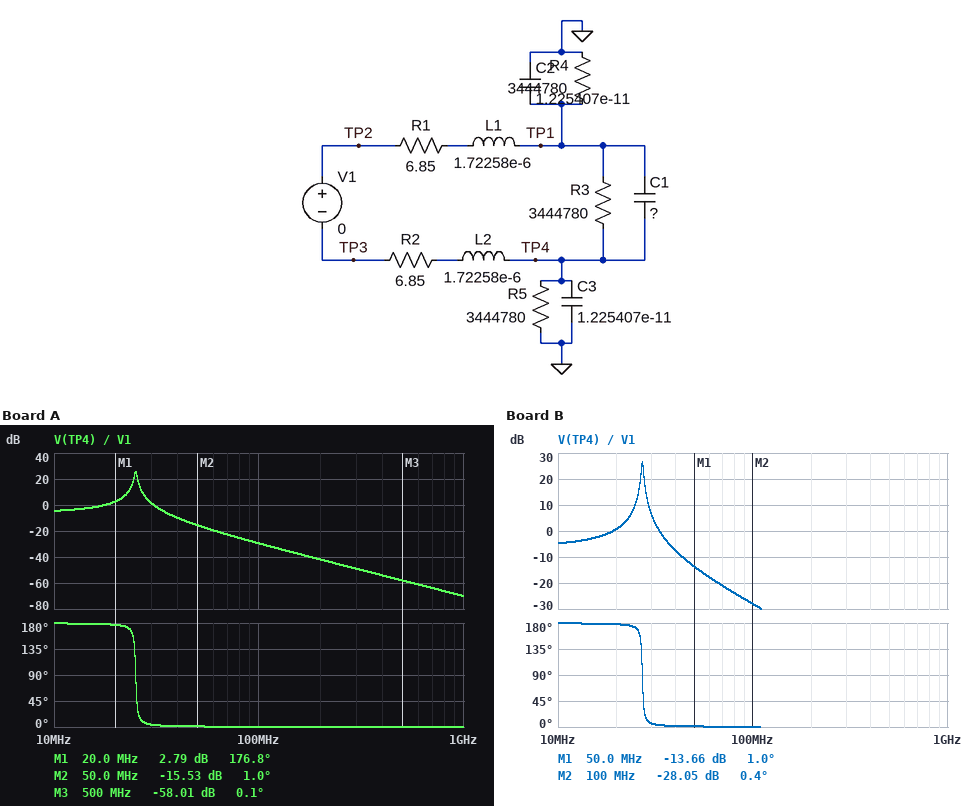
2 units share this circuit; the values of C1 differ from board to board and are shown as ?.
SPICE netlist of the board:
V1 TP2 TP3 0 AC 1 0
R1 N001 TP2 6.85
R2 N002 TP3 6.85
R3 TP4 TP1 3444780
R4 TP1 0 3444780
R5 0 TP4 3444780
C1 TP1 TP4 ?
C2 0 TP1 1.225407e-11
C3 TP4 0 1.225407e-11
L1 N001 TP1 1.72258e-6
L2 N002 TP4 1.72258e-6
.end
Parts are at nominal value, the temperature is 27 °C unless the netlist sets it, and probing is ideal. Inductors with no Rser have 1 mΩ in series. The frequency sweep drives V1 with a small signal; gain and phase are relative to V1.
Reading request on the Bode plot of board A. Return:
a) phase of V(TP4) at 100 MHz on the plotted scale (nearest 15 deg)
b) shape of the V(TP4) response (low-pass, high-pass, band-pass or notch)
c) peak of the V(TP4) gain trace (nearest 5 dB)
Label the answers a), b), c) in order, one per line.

a) 0 deg
b) band-pass
c) 25 dB
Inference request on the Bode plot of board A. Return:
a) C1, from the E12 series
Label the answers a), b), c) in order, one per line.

a) 5.6 pF
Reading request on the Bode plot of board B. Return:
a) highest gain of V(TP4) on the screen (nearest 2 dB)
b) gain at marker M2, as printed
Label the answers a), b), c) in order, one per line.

a) 26 dB
b) -28.05 dB
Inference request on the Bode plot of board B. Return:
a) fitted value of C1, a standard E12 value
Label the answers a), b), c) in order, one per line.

a) 3.9 pF
